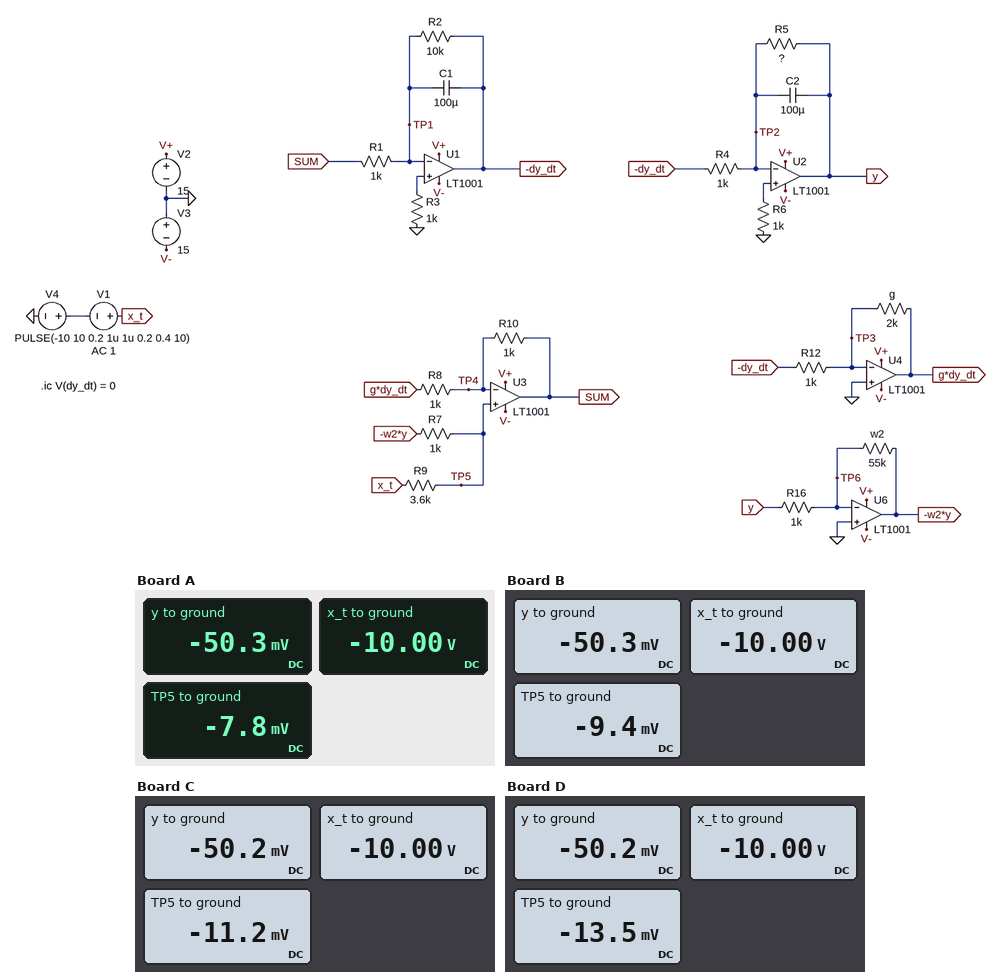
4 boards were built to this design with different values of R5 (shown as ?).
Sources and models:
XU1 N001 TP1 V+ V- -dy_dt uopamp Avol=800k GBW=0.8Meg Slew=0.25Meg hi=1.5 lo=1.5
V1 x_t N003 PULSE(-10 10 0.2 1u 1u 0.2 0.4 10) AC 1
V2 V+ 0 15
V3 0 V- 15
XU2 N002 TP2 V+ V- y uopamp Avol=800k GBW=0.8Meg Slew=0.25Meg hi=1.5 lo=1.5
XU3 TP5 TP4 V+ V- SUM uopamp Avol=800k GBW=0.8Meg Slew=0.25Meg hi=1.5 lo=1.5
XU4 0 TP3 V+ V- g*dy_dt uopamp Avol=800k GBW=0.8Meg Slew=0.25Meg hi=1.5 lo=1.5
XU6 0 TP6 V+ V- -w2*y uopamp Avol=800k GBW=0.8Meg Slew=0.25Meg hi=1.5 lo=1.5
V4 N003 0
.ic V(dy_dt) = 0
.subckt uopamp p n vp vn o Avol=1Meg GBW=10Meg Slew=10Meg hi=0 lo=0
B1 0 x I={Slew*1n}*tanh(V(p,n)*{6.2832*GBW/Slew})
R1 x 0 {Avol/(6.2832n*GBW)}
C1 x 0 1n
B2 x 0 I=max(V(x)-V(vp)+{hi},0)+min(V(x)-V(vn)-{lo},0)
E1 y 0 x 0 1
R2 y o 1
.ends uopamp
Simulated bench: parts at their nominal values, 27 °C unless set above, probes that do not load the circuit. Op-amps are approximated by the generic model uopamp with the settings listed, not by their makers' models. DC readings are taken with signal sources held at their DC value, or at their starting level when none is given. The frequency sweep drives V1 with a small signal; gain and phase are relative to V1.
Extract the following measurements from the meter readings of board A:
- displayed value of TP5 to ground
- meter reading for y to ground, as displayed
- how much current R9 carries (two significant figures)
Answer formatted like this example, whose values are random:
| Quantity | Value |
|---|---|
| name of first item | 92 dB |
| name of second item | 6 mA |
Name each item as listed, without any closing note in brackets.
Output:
| Quantity | Value |
|---|---|
| displayed value of TP5 to ground | -7.8 mV |
| meter reading for y to ground, as displayed | -50.3 mV |
| how much current R9 carries | 2.8 mA |
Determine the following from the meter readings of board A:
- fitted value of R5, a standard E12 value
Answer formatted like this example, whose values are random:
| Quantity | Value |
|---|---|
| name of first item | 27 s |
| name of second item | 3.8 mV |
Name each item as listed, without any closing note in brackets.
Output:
| Quantity | Value |
|---|---|
| fitted value of R5, a standard E12 value | 6.8 kΩ |
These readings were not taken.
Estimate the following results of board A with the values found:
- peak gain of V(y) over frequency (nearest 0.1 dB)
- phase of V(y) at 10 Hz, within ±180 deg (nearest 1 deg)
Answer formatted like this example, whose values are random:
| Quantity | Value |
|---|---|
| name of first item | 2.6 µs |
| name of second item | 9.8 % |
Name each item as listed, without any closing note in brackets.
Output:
| Quantity | Value |
|---|---|
| peak gain of V(y) over frequency | -33.5 dB |
| phase of V(y) at 10 Hz, within ±180 deg | -17 deg |
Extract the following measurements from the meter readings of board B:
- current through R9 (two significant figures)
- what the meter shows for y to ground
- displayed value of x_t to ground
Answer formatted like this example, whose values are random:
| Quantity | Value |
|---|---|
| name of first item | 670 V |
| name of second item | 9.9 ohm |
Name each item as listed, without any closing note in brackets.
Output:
| Quantity | Value |
|---|---|
| current through R9 | 2.8 mA |
| what the meter shows for y to ground | -50.3 mV |
| displayed value of x_t to ground | -10.00 V |
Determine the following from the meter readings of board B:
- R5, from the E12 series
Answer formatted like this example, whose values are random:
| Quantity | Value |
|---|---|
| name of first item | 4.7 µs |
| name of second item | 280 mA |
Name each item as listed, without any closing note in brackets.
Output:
| Quantity | Value |
|---|---|
| R5, from the E12 series | 5.6 kΩ |
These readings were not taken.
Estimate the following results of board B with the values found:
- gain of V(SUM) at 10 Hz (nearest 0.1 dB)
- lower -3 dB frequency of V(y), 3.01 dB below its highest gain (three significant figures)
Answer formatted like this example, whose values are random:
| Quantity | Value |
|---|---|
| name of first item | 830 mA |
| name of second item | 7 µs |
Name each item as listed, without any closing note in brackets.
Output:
| Quantity | Value |
|---|---|
| gain of V(SUM) at 10 Hz | -9.1 dB |
| lower -3 dB frequency of V(y), 3.01 dB below its highest gain | 12.6 Hz |
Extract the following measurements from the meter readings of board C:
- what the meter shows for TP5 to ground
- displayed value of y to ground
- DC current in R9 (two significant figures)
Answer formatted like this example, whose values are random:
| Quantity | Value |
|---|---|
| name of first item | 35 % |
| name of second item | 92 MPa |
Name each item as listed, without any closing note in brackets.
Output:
| Quantity | Value |
|---|---|
| what the meter shows for TP5 to ground | -11.2 mV |
| displayed value of y to ground | -50.2 mV |
| DC current in R9 | 2.8 mA |
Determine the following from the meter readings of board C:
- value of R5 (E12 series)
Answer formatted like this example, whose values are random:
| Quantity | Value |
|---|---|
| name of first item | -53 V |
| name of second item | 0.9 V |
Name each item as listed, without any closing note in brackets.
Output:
| Quantity | Value |
|---|---|
| value of R5 | 4.7 kΩ |
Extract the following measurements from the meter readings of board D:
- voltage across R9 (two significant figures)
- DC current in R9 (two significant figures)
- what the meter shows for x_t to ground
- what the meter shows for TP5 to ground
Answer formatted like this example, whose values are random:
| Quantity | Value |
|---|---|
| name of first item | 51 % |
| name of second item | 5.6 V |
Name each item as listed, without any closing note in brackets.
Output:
| Quantity | Value |
|---|---|
| voltage across R9 | 10 V |
| DC current in R9 | 2.8 mA |
| what the meter shows for x_t to ground | -10.00 V |
| what the meter shows for TP5 to ground | -13.5 mV |
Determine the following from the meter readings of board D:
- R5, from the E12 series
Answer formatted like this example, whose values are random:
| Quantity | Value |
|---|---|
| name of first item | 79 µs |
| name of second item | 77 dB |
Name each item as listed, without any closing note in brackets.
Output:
| Quantity | Value |
|---|---|
| R5, from the E12 series | 3.9 kΩ |
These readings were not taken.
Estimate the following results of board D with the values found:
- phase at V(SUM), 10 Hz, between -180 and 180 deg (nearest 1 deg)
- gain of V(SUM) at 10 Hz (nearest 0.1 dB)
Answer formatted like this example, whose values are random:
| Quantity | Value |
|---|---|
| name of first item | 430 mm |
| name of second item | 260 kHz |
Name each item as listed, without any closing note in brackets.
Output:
| Quantity | Value |
|---|---|
| phase at V(SUM), 10 Hz, between -180 and 180 deg | 159 deg |
| gain of V(SUM) at 10 Hz | -9.2 dB |
